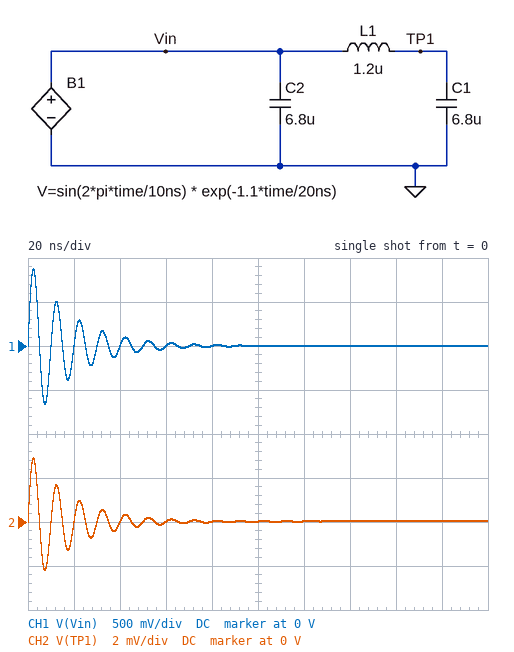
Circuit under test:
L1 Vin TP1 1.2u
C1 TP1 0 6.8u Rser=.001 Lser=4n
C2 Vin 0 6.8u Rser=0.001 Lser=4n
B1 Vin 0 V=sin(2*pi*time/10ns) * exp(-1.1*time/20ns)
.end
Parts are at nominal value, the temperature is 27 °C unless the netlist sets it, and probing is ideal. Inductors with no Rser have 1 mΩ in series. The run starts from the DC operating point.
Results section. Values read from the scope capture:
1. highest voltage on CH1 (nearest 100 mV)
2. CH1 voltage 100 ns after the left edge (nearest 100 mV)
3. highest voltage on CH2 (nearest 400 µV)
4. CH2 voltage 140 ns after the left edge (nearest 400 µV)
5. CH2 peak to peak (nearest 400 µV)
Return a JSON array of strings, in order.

["900 mV", "0 V", "2.8 mV", "0 V", "5.2 mV"]
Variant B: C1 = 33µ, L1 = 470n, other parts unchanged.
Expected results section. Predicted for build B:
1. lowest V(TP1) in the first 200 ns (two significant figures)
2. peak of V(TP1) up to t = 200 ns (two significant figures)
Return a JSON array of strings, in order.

["-5.6 mV", "7.4 mV"]
